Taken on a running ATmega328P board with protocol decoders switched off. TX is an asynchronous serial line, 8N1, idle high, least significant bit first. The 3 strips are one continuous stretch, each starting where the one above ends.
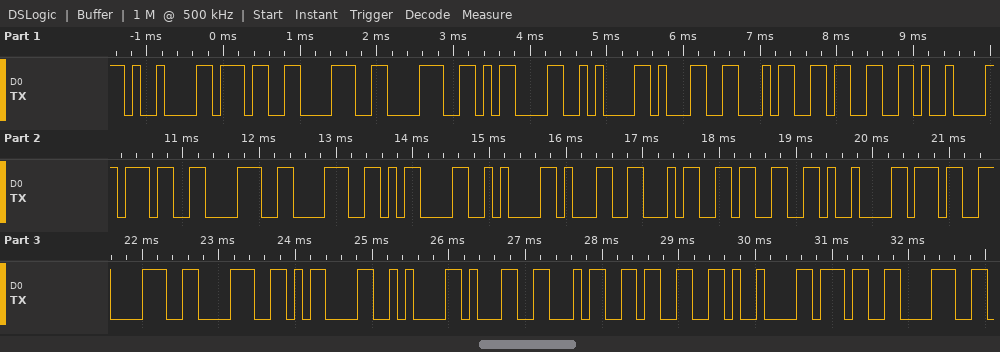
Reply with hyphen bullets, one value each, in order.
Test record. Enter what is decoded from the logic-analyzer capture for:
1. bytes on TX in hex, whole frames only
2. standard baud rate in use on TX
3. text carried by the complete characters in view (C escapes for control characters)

- 09 37 38 38 0D 0A 31 34 33 09 37 38 38 0D 0A 31 34 33 09 37 38 38 0D 0A 31 34 33 09 37 38
- 9600 baud
- "\t788\r\n143\t788\r\n143\t788\r\n143\t78"
